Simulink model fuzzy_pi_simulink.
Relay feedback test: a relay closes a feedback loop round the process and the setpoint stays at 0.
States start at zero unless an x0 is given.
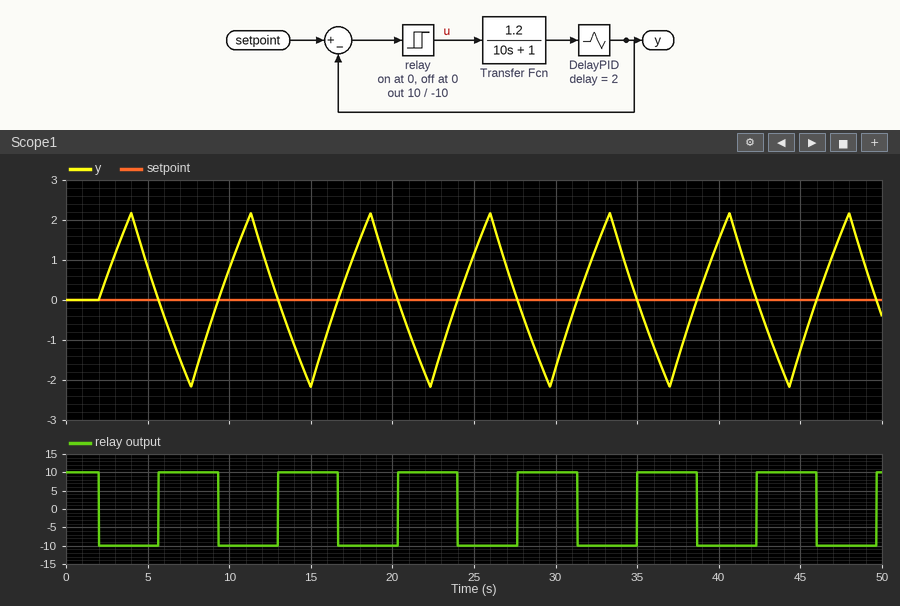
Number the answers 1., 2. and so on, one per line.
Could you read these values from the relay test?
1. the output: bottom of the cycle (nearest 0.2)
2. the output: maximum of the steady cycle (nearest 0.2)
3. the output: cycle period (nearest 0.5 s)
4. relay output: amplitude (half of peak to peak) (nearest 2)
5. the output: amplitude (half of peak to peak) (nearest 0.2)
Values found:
1. -2.2
2. 2.2
3. 7.5 s
4. 10
5. 2.2
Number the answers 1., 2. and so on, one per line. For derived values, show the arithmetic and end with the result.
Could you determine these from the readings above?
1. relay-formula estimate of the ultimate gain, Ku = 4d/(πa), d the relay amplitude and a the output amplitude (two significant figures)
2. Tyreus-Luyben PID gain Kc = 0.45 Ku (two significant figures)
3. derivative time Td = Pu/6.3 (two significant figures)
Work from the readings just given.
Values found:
1. 4 × 10 / (π × 2.2) = 5.8
2. 0.45 × 5.8 = 2.6
3. 7.5 / 6.3 = 1.2 s
